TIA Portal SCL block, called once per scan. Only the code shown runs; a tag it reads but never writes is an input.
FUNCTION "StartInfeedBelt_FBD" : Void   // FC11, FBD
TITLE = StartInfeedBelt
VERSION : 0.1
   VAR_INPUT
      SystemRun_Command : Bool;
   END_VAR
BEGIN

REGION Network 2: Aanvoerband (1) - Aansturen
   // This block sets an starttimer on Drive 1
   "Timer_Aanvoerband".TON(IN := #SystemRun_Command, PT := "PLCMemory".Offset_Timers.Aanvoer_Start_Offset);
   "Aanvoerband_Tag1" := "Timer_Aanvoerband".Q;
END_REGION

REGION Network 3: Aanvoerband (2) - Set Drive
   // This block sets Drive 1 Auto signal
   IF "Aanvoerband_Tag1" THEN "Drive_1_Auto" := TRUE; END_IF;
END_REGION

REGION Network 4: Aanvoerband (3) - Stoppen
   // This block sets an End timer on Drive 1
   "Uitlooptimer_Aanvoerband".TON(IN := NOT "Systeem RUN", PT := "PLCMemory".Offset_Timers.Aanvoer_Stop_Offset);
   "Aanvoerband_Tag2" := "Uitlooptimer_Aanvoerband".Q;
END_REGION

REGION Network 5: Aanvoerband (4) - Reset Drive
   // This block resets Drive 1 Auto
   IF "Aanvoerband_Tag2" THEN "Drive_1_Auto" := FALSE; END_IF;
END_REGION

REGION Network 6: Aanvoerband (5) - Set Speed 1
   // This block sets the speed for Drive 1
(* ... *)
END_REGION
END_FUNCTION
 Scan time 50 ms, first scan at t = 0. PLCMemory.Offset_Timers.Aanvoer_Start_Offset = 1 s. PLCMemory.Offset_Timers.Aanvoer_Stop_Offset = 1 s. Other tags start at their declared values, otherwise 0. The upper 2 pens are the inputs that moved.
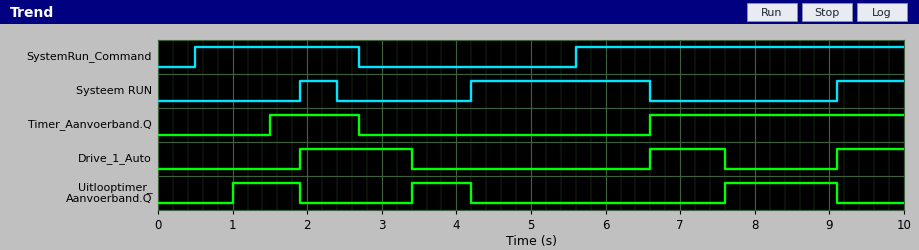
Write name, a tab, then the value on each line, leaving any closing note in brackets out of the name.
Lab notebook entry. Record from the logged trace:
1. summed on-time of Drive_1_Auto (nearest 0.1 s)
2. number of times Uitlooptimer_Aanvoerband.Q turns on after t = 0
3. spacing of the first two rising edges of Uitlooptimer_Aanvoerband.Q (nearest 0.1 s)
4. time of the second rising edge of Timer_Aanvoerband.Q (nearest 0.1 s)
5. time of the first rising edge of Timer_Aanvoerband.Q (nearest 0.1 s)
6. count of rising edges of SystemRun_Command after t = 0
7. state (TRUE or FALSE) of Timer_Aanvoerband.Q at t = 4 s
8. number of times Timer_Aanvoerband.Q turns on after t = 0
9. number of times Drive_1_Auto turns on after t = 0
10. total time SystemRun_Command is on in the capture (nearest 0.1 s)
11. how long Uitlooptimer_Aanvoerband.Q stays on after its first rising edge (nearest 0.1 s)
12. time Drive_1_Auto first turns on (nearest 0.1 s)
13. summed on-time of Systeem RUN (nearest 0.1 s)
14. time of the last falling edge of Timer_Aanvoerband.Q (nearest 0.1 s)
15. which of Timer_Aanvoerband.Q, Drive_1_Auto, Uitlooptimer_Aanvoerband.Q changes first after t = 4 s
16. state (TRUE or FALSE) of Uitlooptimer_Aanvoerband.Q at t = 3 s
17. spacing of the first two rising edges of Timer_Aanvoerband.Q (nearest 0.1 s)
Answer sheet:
summed on-time of Drive_1_Auto	3.4 s
number of times Uitlooptimer_Aanvoerband.Q turns on after t = 0	3
spacing of the first two rising edges of Uitlooptimer_Aanvoerband.Q	2.4 s
time of the second rising edge of Timer_Aanvoerband.Q	6.6 s
time of the first rising edge of Timer_Aanvoerband.Q	1.5 s
count of rising edges of SystemRun_Command after t = 0	2
state (TRUE or FALSE) of Timer_Aanvoerband.Q at t = 4 s	FALSE
number of times Timer_Aanvoerband.Q turns on after t = 0	2
number of times Drive_1_Auto turns on after t = 0	3
total time SystemRun_Command is on in the capture	6.6 s
how long Uitlooptimer_Aanvoerband.Q stays on after its first rising edge	0.9 s
time Drive_1_Auto first turns on	1.9 s
summed on-time of Systeem RUN	3.8 s
time of the last falling edge of Timer_Aanvoerband.Q	2.7 s
which of Timer_Aanvoerband.Q, Drive_1_Auto, Uitlooptimer_Aanvoerband.Q changes first after t = 4 s	Uitlooptimer_Aanvoerband.Q
state (TRUE or FALSE) of Uitlooptimer_Aanvoerband.Q at t = 3 s	FALSE
spacing of the first two rising edges of Timer_Aanvoerband.Q	5.1 s
